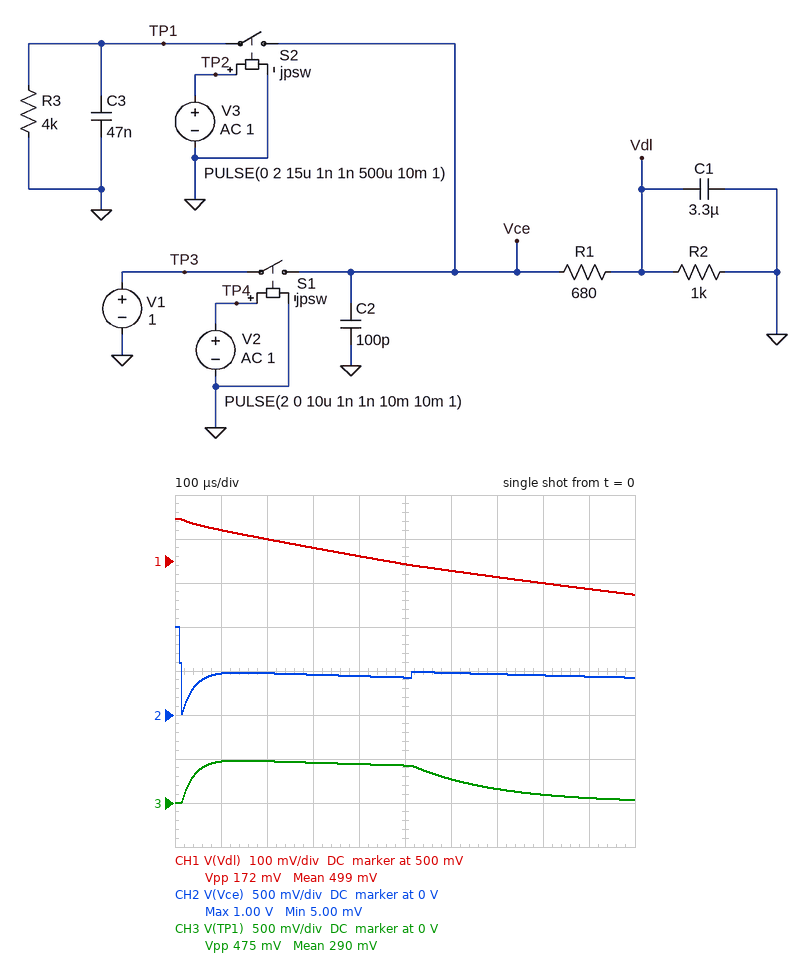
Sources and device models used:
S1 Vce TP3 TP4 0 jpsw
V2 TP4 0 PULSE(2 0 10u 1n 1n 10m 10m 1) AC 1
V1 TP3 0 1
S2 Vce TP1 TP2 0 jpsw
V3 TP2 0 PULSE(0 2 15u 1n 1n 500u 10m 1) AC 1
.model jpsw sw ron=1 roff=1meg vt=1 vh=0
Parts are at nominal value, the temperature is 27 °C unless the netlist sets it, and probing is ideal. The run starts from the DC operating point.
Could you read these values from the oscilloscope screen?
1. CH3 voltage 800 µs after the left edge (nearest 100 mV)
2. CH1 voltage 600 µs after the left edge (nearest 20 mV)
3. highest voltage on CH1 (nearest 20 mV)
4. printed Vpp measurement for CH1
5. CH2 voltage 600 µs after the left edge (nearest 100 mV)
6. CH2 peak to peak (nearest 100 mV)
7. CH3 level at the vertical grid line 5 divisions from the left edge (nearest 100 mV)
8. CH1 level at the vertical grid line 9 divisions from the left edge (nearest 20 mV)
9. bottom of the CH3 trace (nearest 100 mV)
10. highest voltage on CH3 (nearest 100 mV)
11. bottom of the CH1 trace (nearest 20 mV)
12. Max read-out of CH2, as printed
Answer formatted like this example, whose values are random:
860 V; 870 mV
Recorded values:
100 mV; 480 mV; 600 mV; 172 mV; 500 mV; 1.0 V; 400 mV; 440 mV; 0 V; 500 mV; 420 mV; 1.00 V
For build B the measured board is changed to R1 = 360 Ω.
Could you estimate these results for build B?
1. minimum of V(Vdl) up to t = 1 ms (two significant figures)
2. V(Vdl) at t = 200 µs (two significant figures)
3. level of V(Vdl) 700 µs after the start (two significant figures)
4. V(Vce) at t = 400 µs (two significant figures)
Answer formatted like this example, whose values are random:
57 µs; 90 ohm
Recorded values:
520 mV; 680 mV; 570 mV; 580 mV
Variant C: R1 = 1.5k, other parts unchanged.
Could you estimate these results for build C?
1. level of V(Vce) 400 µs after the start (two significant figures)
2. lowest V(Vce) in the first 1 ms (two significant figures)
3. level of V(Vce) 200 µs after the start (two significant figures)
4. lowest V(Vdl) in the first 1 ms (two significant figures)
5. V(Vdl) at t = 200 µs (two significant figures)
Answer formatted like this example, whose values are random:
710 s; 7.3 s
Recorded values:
260 mV; 5.0 mV; 270 mV; 290 mV; 370 mV
